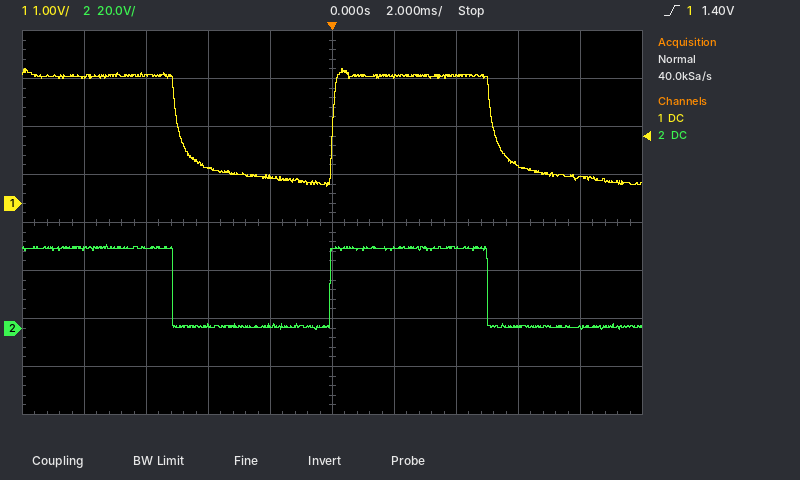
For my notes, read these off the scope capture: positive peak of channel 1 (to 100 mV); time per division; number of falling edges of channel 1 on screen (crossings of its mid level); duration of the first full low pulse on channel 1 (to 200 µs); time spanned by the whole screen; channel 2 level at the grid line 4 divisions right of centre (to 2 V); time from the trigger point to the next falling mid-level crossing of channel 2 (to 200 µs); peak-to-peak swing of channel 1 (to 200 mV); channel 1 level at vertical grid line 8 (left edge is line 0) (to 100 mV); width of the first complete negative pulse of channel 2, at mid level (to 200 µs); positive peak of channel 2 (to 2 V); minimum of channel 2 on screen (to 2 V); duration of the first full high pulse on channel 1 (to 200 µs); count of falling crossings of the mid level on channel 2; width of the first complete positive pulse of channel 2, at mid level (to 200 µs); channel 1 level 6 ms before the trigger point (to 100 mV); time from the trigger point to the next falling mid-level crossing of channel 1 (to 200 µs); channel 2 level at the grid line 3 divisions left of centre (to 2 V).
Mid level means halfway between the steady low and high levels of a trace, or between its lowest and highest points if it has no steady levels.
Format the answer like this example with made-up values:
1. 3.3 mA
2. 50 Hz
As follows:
1. 2.8 V
2. 2 ms
3. 2
4. 5.0 ms
5. 20 ms
6. 0 V
7. 5.0 ms
8. 2.4 V
9. 800 mV
10. 5.0 ms
11. 34 V
12. 0 V
13. 5.2 ms
14. 2
15. 5.0 ms
16. 2.7 V
17. 5.2 ms
18. 34 V
